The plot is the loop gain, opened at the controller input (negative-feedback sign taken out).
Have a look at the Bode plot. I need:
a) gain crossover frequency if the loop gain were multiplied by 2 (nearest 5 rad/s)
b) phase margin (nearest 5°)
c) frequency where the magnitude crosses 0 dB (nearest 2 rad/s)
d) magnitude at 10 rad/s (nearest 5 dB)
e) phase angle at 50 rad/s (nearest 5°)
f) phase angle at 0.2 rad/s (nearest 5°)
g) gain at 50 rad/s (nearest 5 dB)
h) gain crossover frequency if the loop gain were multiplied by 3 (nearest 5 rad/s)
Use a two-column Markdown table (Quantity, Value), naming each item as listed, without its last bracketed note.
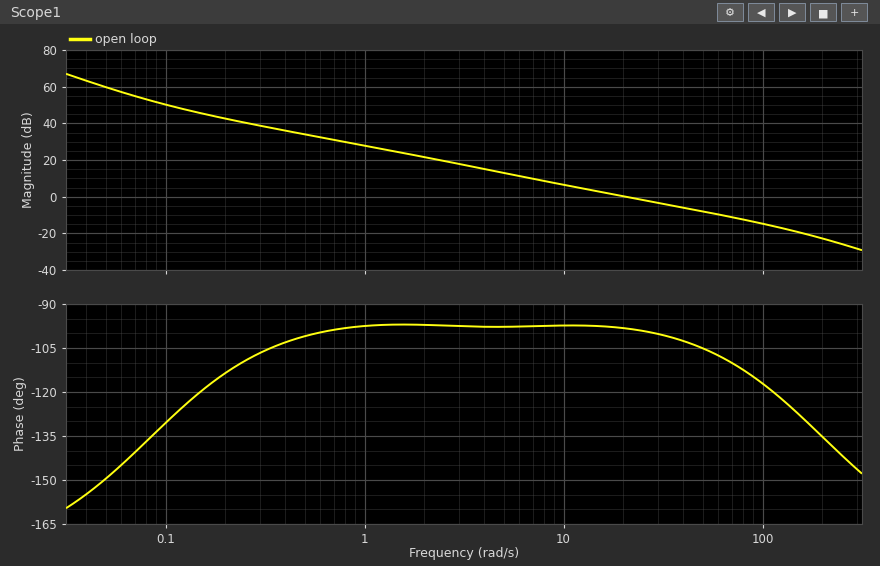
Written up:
| Quantity | Value |
|---|---|
| gain crossover frequency if the loop gain were multiplied by 2 | 40 rad/s |
| phase margin | 80° |
| frequency where the magnitude crosses 0 dB | 20 rad/s |
| magnitude at 10 rad/s | 5 dB |
| phase angle at 50 rad/s | -105° |
| phase angle at 0.2 rad/s | -115° |
| gain at 50 rad/s | -10 dB |
| gain crossover frequency if the loop gain were multiplied by 3 | 60 rad/s |
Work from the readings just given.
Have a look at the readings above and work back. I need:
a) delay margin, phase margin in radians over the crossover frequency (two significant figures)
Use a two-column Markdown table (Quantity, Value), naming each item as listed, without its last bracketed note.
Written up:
| Quantity | Value |
|---|---|
| delay margin, phase margin in radians over the crossover frequency | 0.070 s |
